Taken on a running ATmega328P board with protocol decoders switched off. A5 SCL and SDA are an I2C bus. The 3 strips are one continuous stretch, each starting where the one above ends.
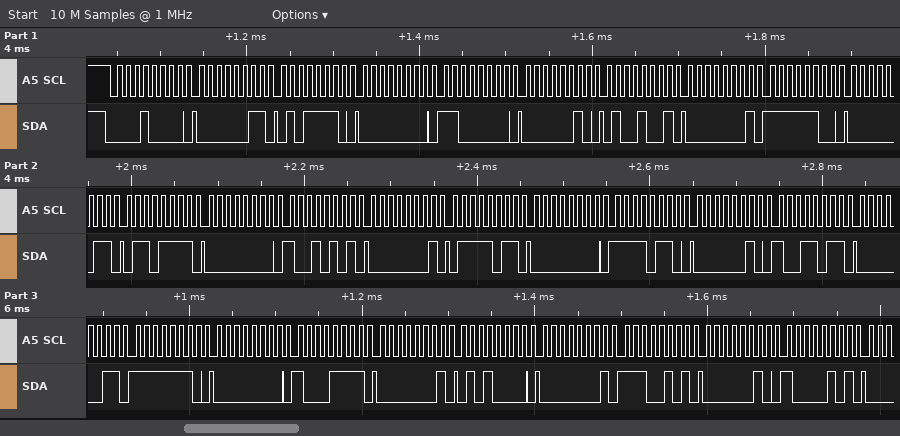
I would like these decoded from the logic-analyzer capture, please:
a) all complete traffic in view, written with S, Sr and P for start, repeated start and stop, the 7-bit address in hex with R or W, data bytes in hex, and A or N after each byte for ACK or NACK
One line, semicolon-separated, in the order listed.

S 08W A 03 A 5E A 00 A C0 A 02 A 49 A 01 A FC A 03 A 6F A 00 A 95 A 01 A 7B A 00 A F6 A 02 A 9B A 03 A FE A 00 A 8F A 01 A 50 A 01 A E5 A 02 A 85 A
